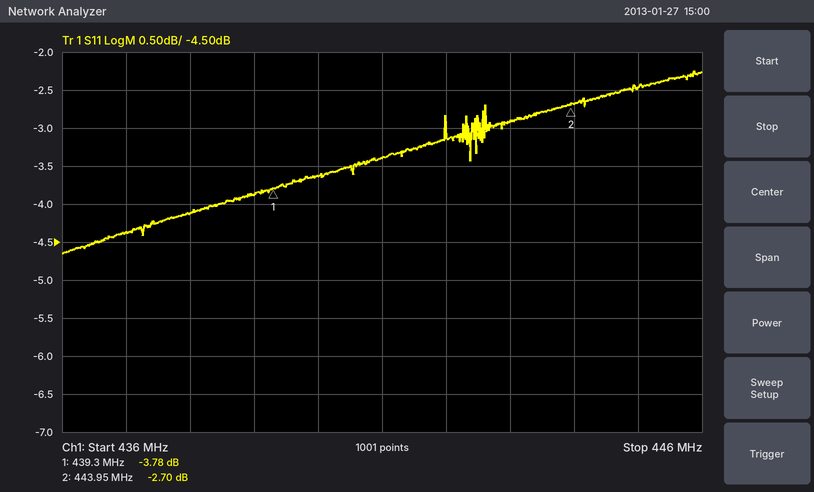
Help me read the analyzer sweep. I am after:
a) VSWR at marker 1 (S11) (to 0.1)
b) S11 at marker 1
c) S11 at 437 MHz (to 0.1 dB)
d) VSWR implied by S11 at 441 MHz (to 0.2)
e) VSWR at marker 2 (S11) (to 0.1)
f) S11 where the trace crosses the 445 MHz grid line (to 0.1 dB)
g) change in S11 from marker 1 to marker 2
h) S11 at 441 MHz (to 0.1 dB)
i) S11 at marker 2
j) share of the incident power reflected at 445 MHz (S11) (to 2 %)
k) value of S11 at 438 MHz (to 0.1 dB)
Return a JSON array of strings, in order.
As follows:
["4.7", "-3.78 dB", "-4.4 dB", "5.2", "6.5", "-2.5 dB", "1.08 dB", "-3.4 dB", "-2.70 dB", "56 %", "-4.1 dB"]
